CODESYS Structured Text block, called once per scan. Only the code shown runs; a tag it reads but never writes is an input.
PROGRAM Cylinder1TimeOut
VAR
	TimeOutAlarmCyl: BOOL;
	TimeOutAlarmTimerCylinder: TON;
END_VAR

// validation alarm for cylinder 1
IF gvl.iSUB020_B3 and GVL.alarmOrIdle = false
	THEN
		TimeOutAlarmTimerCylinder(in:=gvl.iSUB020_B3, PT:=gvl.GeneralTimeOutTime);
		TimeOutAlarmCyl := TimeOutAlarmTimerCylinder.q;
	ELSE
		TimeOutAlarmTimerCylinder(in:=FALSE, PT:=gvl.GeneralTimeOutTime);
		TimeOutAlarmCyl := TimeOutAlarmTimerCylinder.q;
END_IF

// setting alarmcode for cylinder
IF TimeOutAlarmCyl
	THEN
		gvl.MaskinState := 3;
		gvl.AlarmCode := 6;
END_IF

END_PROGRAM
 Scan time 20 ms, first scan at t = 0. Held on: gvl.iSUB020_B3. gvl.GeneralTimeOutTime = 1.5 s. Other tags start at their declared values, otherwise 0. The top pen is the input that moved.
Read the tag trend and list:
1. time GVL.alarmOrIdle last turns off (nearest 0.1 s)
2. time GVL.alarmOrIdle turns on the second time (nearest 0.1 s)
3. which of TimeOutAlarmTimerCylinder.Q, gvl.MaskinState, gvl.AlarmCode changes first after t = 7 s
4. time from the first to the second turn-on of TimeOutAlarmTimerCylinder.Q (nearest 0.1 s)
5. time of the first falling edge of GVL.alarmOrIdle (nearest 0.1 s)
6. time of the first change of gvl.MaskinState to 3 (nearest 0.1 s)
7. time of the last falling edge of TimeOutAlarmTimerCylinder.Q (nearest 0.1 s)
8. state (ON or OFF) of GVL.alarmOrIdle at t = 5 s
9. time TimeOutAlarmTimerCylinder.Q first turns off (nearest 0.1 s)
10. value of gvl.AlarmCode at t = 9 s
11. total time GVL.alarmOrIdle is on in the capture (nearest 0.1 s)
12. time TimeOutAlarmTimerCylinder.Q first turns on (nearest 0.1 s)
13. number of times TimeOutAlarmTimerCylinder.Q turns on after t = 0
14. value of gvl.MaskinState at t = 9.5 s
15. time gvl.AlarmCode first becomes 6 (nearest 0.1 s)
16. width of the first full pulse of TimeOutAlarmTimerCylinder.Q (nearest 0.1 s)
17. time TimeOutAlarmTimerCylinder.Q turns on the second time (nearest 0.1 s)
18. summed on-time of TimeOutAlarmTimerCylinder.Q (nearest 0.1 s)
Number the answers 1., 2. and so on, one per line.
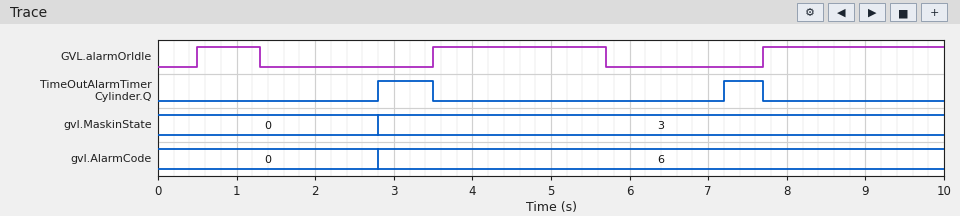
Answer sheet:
1. 5.7 s
2. 3.5 s
3. TimeOutAlarmTimerCylinder.Q
4. 4.4 s
5. 1.3 s
6. 2.8 s
7. 7.7 s
8. ON
9. 3.5 s
10. 6
11. 5.3 s
12. 2.8 s
13. 2
14. 3
15. 2.8 s
16. 0.7 s
17. 7.2 s
18. 1.2 s
